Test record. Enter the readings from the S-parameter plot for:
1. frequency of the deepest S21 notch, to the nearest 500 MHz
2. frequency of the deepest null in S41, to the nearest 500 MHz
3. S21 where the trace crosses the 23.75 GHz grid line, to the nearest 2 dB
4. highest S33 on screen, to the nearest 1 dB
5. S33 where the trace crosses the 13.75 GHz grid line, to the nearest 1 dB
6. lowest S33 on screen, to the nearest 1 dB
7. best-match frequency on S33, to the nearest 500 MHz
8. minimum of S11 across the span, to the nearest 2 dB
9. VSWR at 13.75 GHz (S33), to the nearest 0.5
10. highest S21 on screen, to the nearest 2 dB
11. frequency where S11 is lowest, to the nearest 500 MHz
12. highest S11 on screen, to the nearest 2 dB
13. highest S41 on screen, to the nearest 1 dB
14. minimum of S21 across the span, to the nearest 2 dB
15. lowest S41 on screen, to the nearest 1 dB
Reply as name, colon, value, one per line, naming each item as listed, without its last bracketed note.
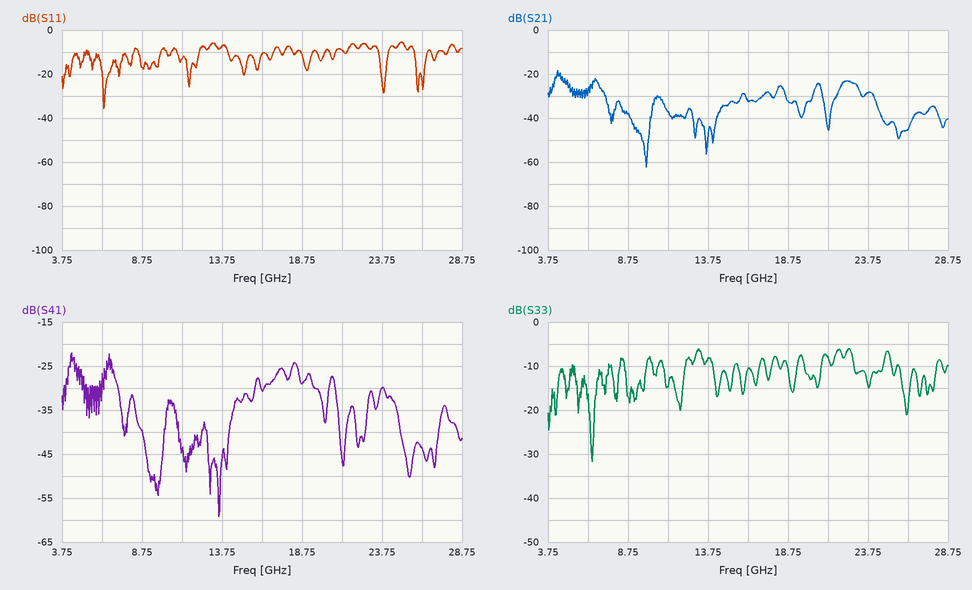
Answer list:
frequency of the deepest S21 notch, to the nearest 500 MHz: 10.0 GHz
frequency of the deepest null in S41, to the nearest 500 MHz: 13.5 GHz
S21 where the trace crosses the 23.75 GHz grid line, to the nearest 2 dB: -28 dB
highest S33 on screen, to the nearest 1 dB: -6 dB
S33 where the trace crosses the 13.75 GHz grid line, to the nearest 1 dB: -8 dB
lowest S33 on screen, to the nearest 1 dB: -32 dB
best-match frequency on S33, to the nearest 500 MHz: 6.5 GHz
minimum of S11 across the span, to the nearest 2 dB: -36 dB
VSWR at 13.75 GHz (S33), to the nearest 0.5: 2.5
highest S21 on screen, to the nearest 2 dB: -18 dB
frequency where S11 is lowest, to the nearest 500 MHz: 6.5 GHz
highest S11 on screen, to the nearest 2 dB: -6 dB
highest S41 on screen, to the nearest 1 dB: -22 dB
minimum of S21 across the span, to the nearest 2 dB: -62 dB
lowest S41 on screen, to the nearest 1 dB: -59 dB
